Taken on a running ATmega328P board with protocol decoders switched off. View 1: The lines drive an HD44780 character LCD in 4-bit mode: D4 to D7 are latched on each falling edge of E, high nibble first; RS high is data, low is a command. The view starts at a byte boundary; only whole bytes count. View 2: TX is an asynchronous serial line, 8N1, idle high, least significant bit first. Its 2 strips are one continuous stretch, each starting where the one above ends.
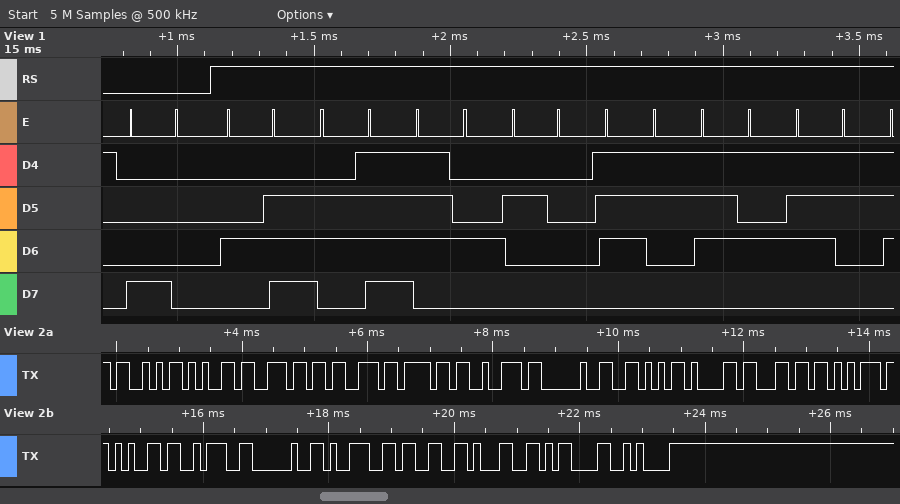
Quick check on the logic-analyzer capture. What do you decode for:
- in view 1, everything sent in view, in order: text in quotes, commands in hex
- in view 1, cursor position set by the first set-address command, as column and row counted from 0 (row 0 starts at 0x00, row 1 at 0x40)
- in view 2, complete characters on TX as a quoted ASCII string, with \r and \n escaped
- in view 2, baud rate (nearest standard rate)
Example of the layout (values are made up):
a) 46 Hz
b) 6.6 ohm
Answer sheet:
a) 0x80 "Not sus"
b) column 0, row 0
c) "Sensor Value: 931\r\n"
d) 9600 baud
